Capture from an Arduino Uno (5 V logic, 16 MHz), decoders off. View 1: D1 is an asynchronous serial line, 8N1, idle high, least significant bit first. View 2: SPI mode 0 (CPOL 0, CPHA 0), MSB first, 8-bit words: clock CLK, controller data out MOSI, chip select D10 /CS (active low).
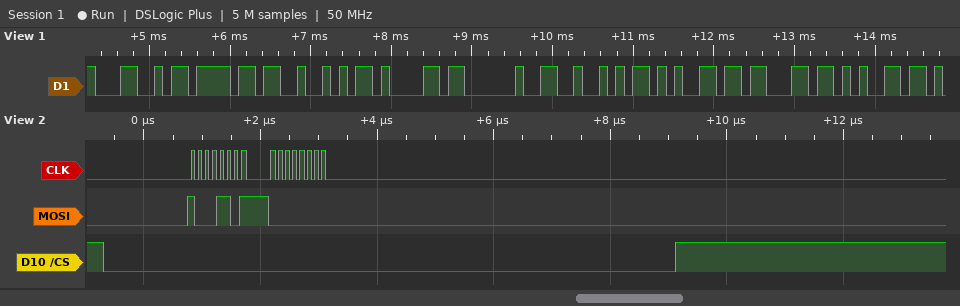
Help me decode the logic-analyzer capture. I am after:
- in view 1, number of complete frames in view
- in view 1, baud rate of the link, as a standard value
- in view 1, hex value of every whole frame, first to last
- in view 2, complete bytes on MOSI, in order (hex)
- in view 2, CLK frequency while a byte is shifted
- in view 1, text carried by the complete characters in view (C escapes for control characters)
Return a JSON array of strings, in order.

["9", "9600 baud", "4C 6F 52 61 20 52 65 63 65", "8D 00", "8 MHz", "\"LoRa Rece\""]
